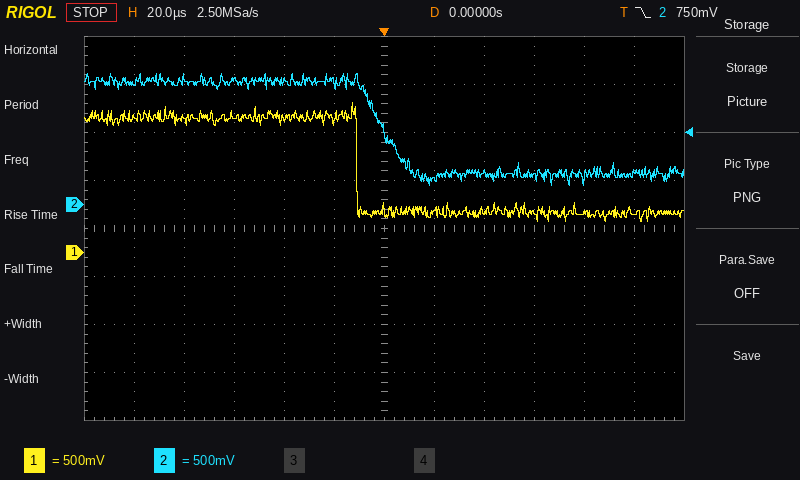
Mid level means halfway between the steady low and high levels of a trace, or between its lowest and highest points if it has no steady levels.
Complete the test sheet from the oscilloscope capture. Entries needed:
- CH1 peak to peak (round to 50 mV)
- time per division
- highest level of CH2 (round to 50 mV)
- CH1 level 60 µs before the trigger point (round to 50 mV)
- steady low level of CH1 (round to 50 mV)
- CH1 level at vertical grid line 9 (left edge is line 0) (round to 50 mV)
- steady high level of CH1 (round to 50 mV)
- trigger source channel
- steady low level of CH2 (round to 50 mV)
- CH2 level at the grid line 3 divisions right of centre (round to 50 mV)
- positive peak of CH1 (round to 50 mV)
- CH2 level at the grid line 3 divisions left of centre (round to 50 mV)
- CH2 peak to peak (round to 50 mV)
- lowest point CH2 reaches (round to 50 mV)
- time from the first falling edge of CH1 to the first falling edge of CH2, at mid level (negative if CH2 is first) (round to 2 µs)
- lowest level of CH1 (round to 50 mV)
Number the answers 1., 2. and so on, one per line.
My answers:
1. 1.25 V
2. 20 µs
3. 1.35 V
4. 1.45 V
5. 400 mV
6. 400 mV
7. 1.40 V
8. CH2
9. 300 mV
10. 300 mV
11. 1.55 V
12. 1.30 V
13. 1.15 V
14. 200 mV
15. +10 µs
16. 300 mV
